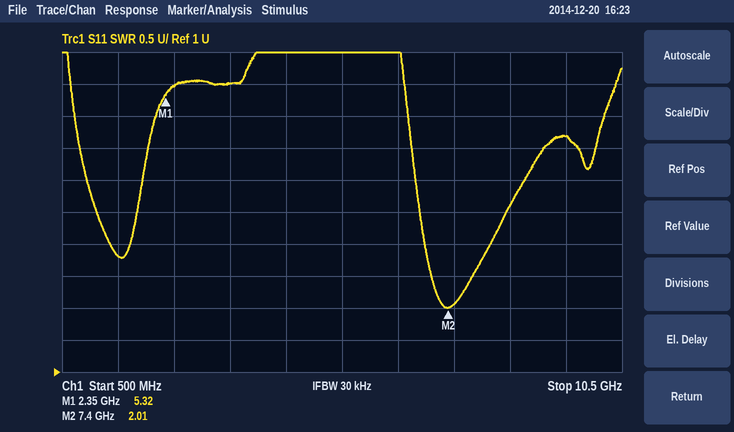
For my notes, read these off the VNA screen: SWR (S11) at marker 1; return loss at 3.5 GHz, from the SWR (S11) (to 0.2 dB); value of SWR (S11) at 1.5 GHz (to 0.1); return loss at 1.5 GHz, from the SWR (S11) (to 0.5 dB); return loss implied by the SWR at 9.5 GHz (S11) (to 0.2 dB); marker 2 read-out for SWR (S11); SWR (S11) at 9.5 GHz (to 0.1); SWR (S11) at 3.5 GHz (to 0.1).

5.32
3.2 dB
2.8
6.5 dB
3.8 dB
2.01
4.7
5.5
